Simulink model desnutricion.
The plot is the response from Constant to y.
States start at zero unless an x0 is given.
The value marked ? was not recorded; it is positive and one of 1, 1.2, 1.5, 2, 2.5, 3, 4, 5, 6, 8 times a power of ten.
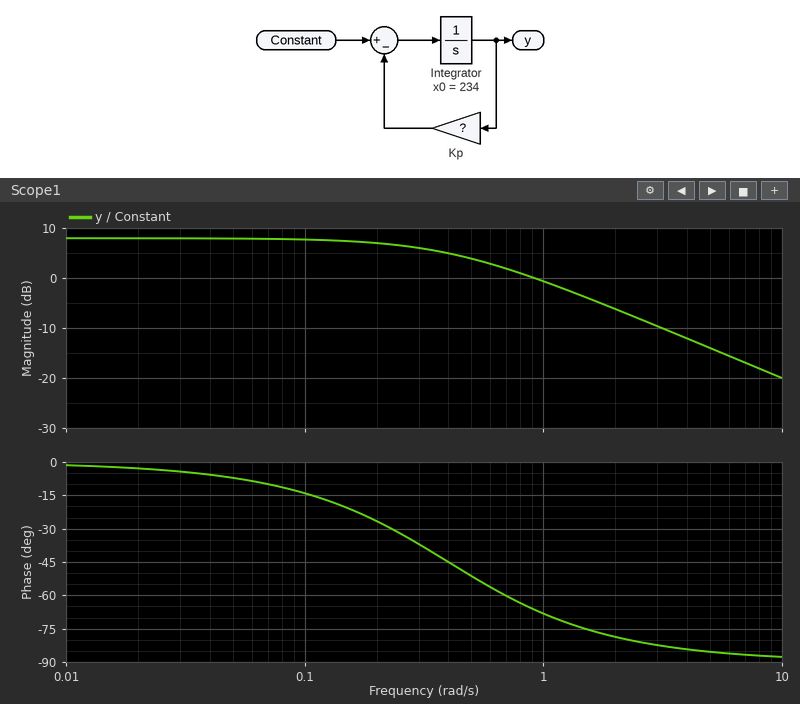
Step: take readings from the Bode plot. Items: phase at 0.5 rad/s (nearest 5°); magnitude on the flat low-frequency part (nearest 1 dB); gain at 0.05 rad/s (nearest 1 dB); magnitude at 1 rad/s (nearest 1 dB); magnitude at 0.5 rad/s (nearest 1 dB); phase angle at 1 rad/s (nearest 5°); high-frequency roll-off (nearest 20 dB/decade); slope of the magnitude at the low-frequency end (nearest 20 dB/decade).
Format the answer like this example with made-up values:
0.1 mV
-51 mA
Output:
-50°
8 dB
8 dB
-1 dB
4 dB
-70°
-20 dB/decade
0 dB/decade
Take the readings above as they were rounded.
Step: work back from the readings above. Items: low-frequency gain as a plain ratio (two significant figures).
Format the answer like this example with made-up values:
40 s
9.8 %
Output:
2.5
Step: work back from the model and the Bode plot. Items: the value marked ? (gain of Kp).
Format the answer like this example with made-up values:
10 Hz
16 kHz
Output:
0.4
